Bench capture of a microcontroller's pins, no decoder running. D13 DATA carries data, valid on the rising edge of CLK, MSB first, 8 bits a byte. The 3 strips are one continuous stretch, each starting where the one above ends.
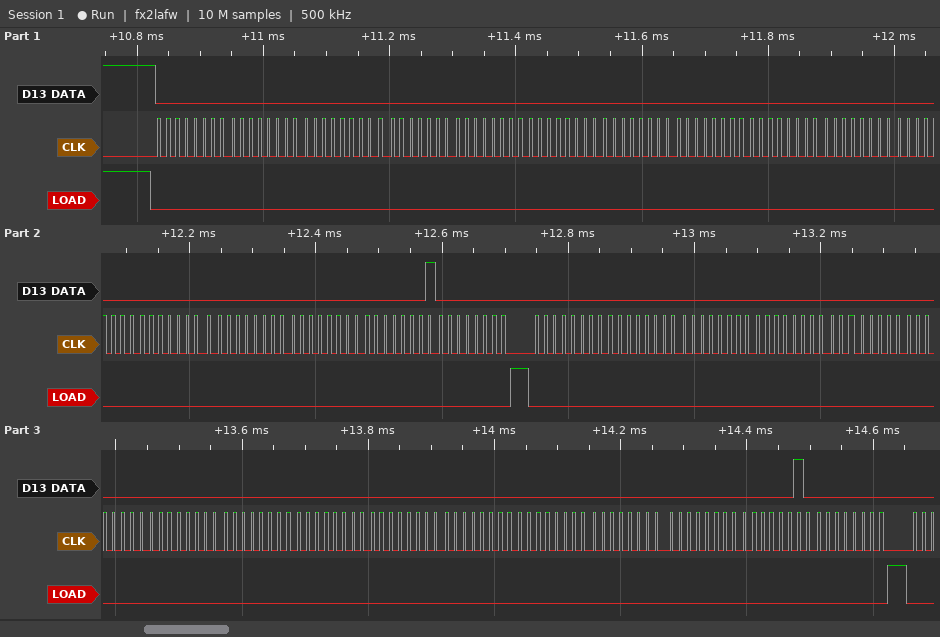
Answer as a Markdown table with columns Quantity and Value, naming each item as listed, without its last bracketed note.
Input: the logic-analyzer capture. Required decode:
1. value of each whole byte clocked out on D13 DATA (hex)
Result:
| Quantity | Value |
|---|---|
| value of each whole byte clocked out on D13 DATA | 00 00 00 00 00 00 00 00 00 00 00 00 00 00 01 00 00 00 00 00 00 00 00 00 00 00 00 00 00 00 02 00 |
